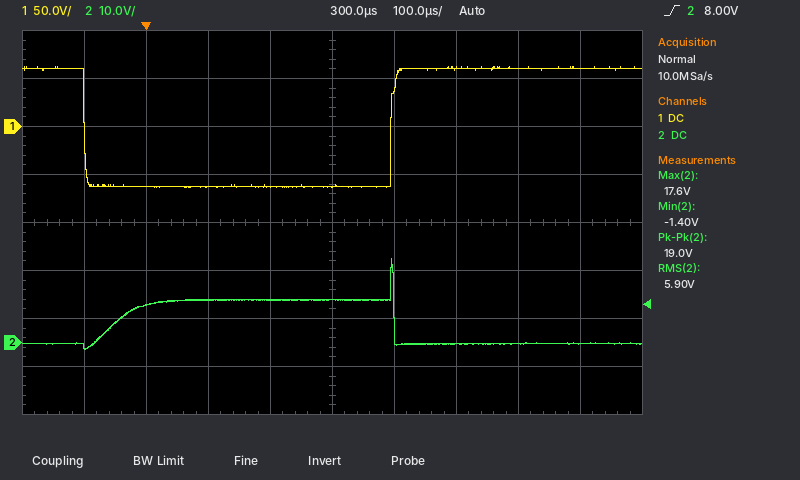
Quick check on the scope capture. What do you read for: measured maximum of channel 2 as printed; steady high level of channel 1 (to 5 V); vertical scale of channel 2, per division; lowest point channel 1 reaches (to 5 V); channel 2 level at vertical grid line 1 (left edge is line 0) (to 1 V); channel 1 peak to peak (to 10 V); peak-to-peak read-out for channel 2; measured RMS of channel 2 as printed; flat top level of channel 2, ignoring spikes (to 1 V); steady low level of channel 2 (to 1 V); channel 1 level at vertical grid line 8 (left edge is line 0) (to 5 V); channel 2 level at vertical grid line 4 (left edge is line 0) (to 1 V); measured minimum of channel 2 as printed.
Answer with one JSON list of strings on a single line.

["17.6 V", "60 V", "10 V", "-65 V", "-1 V", "130 V", "19.0 V", "5.90 V", "9 V", "0 V", "60 V", "9 V", "-1.40 V"]
